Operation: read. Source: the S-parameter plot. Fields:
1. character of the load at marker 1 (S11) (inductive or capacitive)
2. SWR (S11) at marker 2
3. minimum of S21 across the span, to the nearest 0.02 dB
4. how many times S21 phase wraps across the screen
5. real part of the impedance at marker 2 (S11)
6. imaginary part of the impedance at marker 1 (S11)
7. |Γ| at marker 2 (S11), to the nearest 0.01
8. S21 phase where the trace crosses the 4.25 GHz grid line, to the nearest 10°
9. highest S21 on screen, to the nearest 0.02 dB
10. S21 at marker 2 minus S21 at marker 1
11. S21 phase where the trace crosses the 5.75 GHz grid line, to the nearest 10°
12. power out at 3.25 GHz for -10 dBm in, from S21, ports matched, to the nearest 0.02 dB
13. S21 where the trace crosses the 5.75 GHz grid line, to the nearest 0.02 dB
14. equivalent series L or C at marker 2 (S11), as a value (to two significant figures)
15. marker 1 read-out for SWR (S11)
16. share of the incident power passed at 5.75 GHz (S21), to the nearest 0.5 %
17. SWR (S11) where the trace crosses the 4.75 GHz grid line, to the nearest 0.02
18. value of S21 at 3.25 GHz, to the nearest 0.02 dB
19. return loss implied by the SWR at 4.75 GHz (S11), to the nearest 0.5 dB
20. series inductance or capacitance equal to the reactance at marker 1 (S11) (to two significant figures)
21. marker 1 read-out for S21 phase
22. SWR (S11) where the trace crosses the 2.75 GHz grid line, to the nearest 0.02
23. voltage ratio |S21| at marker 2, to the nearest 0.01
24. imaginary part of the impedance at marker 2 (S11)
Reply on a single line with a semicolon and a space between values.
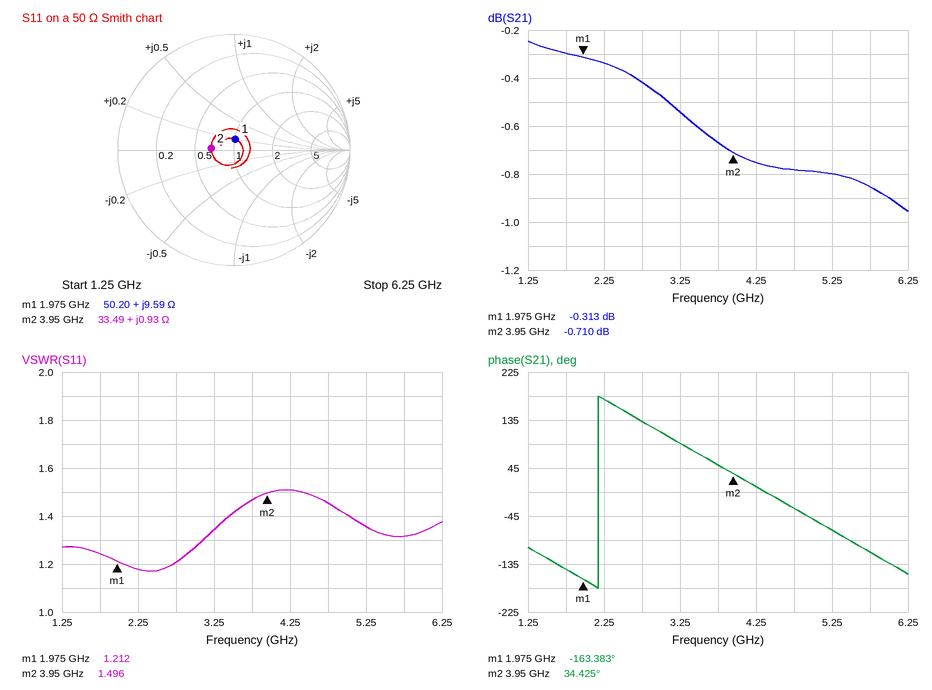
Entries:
inductive; 1.496; -0.96 dB; 1; 33.49 Ω; +9.59 Ω; 0.20; 10°; -0.24 dB; -0.397 dB; -110°; -10.54 dBm; -0.86 dB; 37 pH; 1.212; 82.0 %; 1.46; -0.54 dB; 14.5 dB; 770 pH; -163.383°; 1.20; 0.92; +0.93 Ω
